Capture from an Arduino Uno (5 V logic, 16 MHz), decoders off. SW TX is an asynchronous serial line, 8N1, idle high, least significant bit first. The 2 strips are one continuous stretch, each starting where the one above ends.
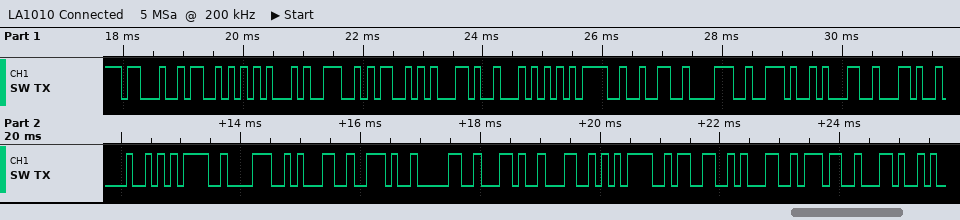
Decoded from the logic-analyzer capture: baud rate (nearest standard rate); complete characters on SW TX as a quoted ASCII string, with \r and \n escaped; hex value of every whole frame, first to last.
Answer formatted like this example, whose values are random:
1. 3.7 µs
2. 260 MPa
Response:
1. 9600 baud
2. "#SENS,T=28.1,H=81.0,L=317,"
3. 23 53 45 4E 53 2C 54 3D 32 38 2E 31 2C 48 3D 38 31 2E 30 2C 4C 3D 33 31 37 2C
